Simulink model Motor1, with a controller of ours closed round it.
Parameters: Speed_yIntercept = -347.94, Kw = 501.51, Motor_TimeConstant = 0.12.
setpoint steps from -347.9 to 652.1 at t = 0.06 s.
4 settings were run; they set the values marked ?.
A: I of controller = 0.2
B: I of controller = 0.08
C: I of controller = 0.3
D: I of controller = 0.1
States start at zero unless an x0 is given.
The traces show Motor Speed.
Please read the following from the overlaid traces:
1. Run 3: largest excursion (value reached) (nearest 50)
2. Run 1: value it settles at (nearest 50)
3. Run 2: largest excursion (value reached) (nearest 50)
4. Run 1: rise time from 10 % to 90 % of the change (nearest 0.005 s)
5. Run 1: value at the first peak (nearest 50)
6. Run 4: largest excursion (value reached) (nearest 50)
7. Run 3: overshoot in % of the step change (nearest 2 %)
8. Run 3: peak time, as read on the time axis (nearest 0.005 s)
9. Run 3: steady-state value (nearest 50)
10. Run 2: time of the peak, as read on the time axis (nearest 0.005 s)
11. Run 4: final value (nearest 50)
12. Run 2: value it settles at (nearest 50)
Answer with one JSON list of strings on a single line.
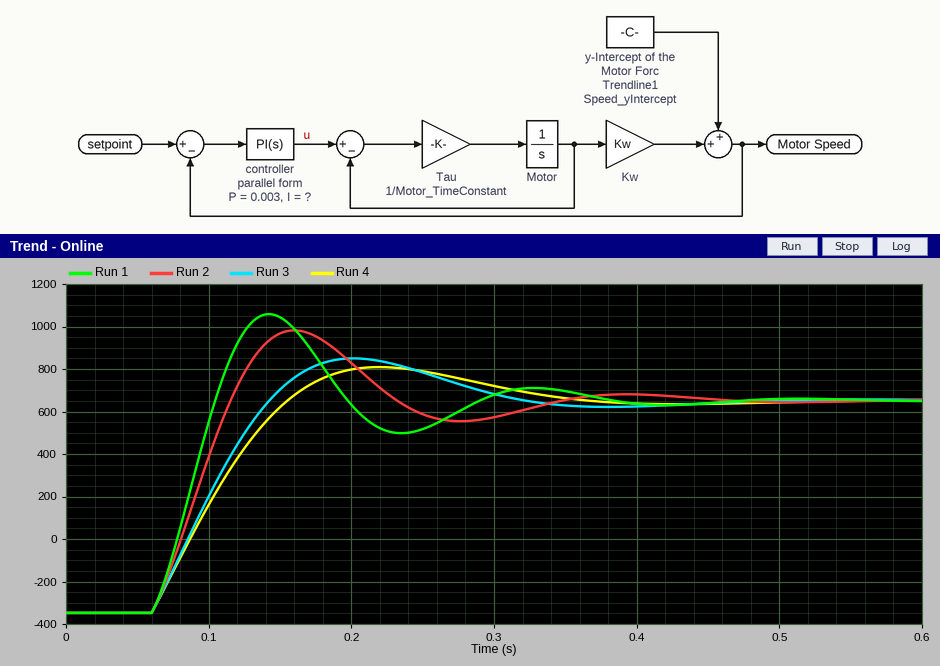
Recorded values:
["850", "650", "1000", "0.035 s", "1050", "800", "20 %", "0.200 s", "650", "0.160 s", "650", "650"]
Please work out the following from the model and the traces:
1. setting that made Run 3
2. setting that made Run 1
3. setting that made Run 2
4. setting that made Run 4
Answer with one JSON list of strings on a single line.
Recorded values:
["D", "C", "A", "B"]
